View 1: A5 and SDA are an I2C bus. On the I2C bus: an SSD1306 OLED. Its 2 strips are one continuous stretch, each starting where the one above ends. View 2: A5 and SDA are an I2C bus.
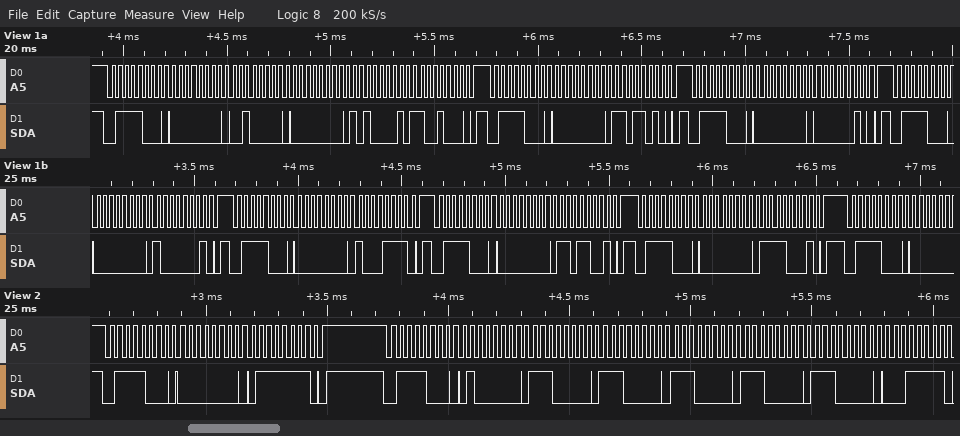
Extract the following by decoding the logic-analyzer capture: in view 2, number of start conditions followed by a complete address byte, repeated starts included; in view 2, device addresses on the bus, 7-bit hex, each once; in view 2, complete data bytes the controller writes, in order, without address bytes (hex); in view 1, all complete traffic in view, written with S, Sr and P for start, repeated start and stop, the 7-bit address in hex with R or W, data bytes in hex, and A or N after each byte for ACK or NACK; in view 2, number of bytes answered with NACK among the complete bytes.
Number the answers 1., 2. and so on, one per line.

1. 2
2. 0x3C
3. 00 7F 40 E0 E0 E0 E0 E0 1F
4. S 3CW A 00 A 20 A 00 A A1 A C8 A P S 3CW A 00 A DA A P S 3CW A 00 A 02 A P S 3CW A 00 A 81 A P S 3CW A 00 A 8F A P S 3CW A 00 A D9 A P S 3CW A 00 A F1 A P S 3CW A
5. 0
